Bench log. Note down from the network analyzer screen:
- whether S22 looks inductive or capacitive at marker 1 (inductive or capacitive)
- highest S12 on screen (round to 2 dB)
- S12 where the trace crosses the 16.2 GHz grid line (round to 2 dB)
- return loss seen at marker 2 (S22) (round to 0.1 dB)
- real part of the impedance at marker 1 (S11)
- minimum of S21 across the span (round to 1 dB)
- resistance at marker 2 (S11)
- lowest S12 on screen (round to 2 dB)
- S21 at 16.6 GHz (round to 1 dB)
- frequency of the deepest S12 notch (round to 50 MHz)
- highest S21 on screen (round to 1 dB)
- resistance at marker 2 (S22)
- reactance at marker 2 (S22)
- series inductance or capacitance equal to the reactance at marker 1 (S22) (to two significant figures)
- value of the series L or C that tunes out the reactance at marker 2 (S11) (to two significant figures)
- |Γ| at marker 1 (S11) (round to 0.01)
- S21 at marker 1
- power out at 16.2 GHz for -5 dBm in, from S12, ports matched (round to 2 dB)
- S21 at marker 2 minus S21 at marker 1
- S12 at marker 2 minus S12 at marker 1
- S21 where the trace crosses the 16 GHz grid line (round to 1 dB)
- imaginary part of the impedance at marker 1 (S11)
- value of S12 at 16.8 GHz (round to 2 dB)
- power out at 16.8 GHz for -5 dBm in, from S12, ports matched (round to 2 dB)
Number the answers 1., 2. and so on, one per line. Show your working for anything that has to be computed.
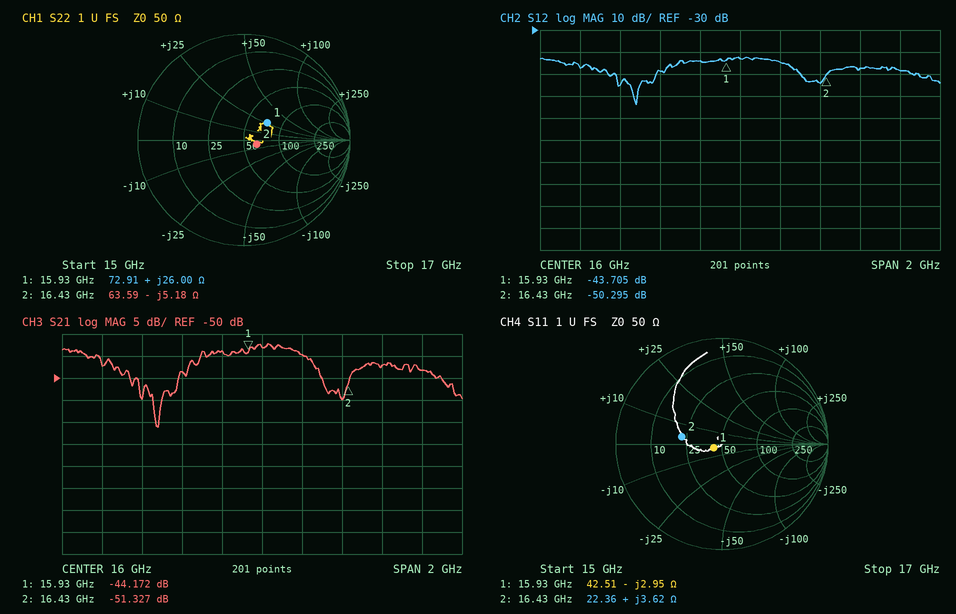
1. inductive
2. -42 dB
3. -44 dB
4. 17.9 dB
5. 42.51 Ω
6. -61 dB
7. 22.36 Ω
8. -64 dB
9. -47 dB
10. 15.50 GHz
11. -42 dB
12. 63.59 Ω
13. -5.18 Ω
14. L = 26 Ω/(2π × 15.93 GHz) ≈ 260 pH
15. C = 1/(2π × 16.43 GHz × 3.62 Ω) ≈ 2.7 pF
16. 0.09
17. -44.172 dB
18. -5 dBm + (-44 dB) = -50 dBm
19. -51.327 − (-44.172) = -7.155 dB
20. -50.295 − (-43.705) = -6.590 dB
21. -43 dB
22. -2.95 Ω
23. -48 dB
24. -5 dBm + (-48 dB) = -54 dBm
